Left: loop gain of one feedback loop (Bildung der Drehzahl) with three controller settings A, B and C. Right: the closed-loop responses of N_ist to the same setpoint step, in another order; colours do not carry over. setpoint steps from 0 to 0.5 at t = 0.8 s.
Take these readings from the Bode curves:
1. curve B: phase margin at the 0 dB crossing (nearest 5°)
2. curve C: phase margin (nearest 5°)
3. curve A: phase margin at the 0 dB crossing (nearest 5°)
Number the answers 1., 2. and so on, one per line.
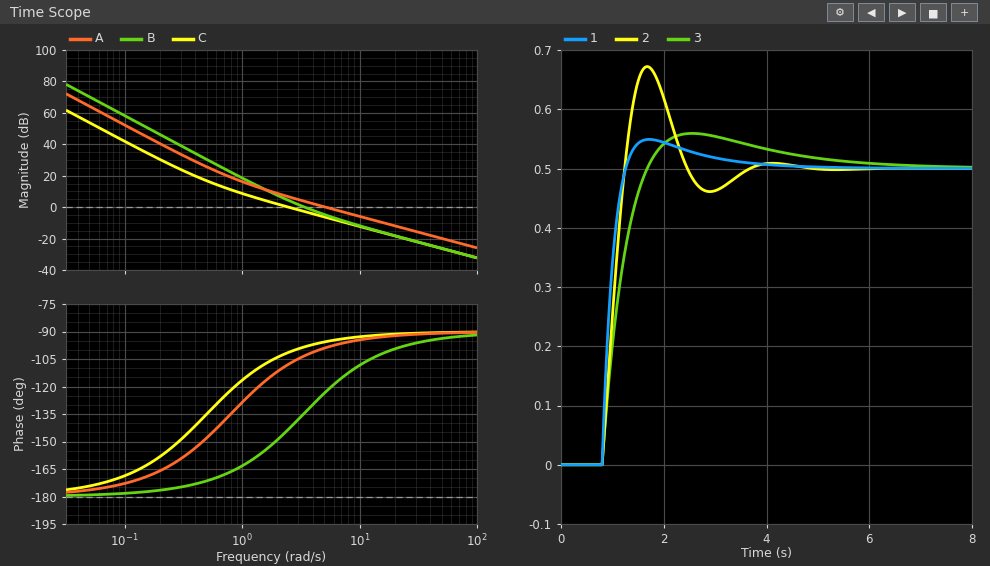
1. 45°
2. 80°
3. 80°
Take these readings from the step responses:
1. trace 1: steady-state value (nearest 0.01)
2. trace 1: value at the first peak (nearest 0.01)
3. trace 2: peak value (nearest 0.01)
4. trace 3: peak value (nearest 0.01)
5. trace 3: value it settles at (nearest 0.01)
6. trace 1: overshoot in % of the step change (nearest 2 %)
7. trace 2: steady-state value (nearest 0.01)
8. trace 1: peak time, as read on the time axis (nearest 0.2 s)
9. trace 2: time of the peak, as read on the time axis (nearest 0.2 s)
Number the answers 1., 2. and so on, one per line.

1. 0.50
2. 0.55
3. 0.67
4. 0.56
5. 0.50
6. 10 %
7. 0.50
8. 1.8 s
9. 1.6 s
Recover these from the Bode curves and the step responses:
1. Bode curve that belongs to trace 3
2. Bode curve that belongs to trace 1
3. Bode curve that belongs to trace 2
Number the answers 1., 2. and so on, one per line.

1. C
2. A
3. B
